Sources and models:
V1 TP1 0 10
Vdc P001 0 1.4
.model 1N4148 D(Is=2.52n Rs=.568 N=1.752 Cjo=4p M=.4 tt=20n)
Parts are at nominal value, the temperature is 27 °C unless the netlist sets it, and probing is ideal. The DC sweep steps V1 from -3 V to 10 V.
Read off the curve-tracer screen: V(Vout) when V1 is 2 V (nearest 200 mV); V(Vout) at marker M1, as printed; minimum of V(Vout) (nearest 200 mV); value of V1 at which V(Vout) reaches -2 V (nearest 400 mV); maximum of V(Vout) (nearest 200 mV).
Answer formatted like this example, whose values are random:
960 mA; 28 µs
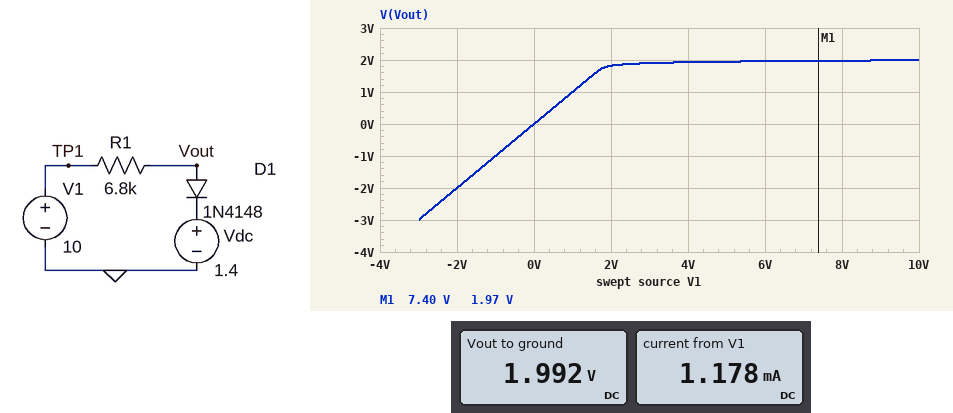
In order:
1.8 V; 1.97 V; -3.0 V; -2.0 V; 2.0 V
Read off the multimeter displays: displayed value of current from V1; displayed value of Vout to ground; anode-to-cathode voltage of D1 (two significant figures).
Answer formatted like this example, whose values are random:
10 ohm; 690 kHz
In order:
1.178 mA; 1.992 V; 590 mV
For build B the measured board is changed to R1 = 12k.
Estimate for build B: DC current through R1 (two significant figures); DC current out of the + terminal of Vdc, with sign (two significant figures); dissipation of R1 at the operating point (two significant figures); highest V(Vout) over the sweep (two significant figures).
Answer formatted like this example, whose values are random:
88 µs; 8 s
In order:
670 µA; -670 µA; 5.4 mW; 2.0 V
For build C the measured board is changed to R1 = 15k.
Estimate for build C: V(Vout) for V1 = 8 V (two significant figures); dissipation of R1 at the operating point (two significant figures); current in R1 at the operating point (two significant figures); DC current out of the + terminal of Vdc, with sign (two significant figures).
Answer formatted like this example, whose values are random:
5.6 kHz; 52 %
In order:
1.9 V; 4.3 mW; 540 µA; -540 µA
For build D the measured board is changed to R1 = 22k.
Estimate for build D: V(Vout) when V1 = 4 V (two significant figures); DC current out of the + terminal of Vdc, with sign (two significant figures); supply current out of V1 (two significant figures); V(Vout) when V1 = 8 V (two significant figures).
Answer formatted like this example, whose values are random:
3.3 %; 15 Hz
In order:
1.9 V; -370 µA; 370 µA; 1.9 V
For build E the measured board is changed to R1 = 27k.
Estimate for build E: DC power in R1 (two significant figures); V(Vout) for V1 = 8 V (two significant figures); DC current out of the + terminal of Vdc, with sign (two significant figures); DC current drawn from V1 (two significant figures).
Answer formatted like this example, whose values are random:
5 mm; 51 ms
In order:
2.4 mW; 1.9 V; -300 µA; 300 µA
